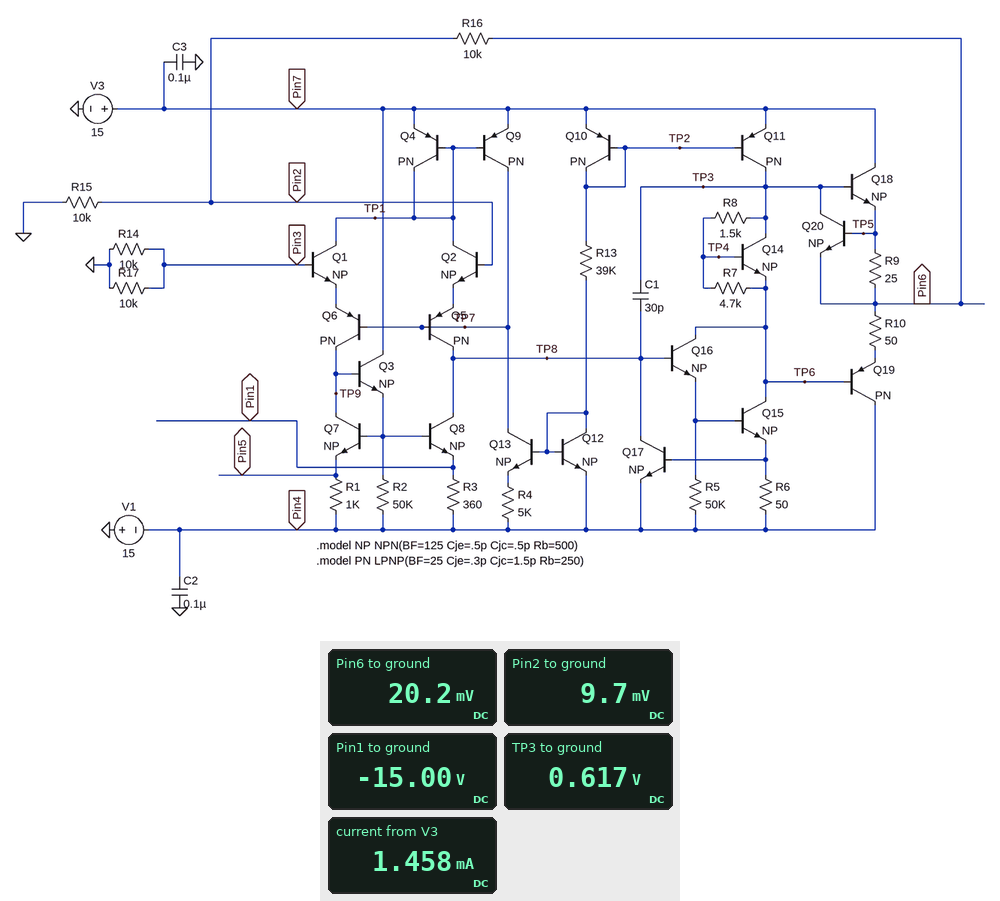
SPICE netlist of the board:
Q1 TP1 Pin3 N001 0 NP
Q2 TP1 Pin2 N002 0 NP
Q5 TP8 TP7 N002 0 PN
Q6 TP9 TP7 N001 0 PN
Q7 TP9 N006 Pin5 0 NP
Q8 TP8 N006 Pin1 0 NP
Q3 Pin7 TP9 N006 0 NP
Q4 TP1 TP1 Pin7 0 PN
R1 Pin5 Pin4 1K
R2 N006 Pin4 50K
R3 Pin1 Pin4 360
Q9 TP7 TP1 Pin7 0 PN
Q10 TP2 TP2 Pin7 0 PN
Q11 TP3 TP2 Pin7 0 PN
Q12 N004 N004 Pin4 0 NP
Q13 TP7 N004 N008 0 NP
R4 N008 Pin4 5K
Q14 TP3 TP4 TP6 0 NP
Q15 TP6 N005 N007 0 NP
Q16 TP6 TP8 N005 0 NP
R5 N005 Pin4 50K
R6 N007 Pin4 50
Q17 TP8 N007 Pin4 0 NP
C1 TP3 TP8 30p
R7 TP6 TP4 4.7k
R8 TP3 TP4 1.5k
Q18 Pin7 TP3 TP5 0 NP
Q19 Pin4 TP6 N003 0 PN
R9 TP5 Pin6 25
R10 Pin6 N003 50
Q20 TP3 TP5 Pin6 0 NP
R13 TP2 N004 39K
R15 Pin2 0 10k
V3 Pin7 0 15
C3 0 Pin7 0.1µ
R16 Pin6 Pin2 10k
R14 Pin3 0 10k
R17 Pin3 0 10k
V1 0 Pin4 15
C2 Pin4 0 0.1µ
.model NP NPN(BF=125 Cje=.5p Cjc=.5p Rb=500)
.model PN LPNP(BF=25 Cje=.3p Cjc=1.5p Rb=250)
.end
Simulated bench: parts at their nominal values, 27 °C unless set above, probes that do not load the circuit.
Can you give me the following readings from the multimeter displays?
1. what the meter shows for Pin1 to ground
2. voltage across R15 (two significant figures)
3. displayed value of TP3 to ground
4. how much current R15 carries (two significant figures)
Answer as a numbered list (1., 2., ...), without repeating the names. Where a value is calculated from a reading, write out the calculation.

1. -15.00 V
2. 9.7 mV = 9.7 mV
3. 0.617 V
4. (9.7 mV) / 10 kΩ = 970 nA
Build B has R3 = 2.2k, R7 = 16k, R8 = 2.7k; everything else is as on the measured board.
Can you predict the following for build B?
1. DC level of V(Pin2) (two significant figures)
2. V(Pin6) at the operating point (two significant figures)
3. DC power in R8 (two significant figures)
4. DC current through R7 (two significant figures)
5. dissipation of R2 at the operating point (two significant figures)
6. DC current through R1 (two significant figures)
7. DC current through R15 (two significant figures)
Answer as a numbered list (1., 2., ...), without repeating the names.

1. -14 mV
2. -28 mV
3. 7.5 µW
4. 48 µA
5. 8.9 µW
6. 11 µA
7. 1.4 µA
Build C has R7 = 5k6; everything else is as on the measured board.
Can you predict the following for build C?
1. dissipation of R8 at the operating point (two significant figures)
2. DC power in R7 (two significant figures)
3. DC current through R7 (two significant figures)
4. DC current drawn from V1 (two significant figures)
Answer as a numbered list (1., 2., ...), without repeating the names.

1. 29 µW
2. 100 µW
3. 140 µA
4. 1.5 mA
